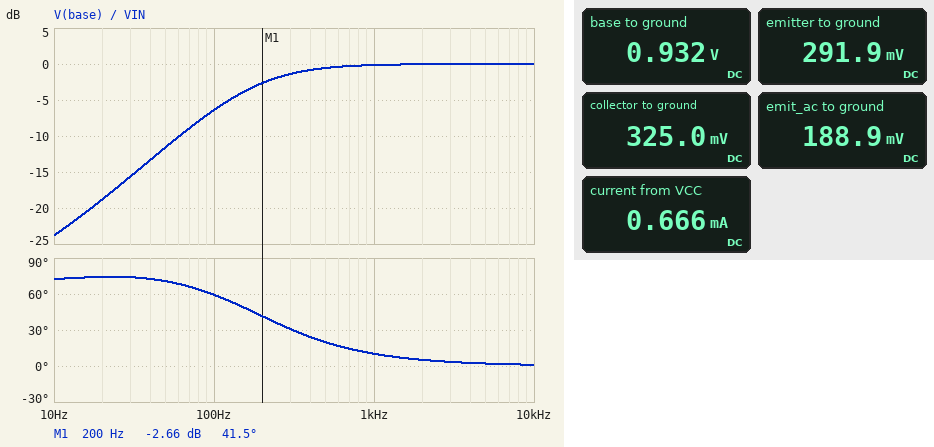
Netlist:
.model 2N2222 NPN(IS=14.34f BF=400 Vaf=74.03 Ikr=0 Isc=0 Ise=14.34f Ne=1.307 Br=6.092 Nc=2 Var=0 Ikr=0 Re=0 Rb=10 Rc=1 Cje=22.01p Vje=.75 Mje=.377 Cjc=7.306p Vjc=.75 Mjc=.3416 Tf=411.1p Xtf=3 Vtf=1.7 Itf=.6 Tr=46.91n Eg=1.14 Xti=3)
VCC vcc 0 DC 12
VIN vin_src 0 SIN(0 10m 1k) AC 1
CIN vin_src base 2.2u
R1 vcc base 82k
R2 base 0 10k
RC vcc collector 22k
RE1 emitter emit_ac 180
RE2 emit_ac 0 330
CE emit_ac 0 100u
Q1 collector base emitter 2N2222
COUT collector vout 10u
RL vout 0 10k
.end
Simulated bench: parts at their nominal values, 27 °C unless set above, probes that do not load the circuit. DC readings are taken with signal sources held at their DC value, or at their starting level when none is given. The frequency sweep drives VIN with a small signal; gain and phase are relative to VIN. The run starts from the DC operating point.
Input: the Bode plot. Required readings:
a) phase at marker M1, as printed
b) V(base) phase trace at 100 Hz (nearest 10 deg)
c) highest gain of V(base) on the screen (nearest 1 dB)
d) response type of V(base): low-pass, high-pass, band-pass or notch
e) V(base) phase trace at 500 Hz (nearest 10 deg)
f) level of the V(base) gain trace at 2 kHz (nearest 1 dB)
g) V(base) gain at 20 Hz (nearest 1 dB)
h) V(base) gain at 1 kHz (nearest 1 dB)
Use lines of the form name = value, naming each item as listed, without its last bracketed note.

phase at marker M1, as printed = 41.5 deg
V(base) phase trace at 100 Hz = 60 deg
highest gain of V(base) on the screen = 0 dB
response type of V(base): low-pass, high-pass, band-pass or notch = high-pass
V(base) phase trace at 500 Hz = 20 deg
level of the V(base) gain trace at 2 kHz = 0 dB
V(base) gain at 20 Hz = -19 dB
V(base) gain at 1 kHz = 0 dB
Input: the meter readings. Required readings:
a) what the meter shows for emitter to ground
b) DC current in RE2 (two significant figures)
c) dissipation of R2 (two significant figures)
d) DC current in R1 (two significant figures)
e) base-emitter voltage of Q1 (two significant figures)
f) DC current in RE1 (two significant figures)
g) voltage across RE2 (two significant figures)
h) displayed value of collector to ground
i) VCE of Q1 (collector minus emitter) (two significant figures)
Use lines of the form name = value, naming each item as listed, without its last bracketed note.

what the meter shows for emitter to ground = 291.9 mV
DC current in RE2 = 570 µA
dissipation of R2 = 87 µW
DC current in R1 = 130 µA
base-emitter voltage of Q1 = 640 mV
DC current in RE1 = 570 µA
voltage across RE2 = 190 mV
displayed value of collector to ground = 325.0 mV
VCE of Q1 (collector minus emitter) = 33 mV
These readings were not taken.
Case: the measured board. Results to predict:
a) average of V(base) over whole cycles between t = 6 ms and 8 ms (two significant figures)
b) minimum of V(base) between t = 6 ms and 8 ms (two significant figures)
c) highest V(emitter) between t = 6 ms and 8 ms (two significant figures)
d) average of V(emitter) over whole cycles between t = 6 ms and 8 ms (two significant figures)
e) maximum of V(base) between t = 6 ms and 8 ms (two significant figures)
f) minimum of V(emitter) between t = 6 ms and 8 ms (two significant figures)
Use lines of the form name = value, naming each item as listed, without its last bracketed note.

average of V(base) over whole cycles between t = 6 ms and 8 ms = 930 mV
minimum of V(base) between t = 6 ms and 8 ms = 920 mV
highest V(emitter) between t = 6 ms and 8 ms = 300 mV
average of V(emitter) over whole cycles between t = 6 ms and 8 ms = 290 mV
maximum of V(base) between t = 6 ms and 8 ms = 940 mV
minimum of V(emitter) between t = 6 ms and 8 ms = 290 mV
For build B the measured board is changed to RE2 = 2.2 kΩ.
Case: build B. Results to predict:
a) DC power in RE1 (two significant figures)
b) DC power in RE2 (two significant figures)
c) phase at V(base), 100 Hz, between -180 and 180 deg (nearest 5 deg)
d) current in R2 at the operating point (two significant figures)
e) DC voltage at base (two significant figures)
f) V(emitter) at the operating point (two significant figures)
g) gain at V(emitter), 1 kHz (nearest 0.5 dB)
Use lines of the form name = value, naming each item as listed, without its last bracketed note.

DC power in RE1 = 15 µW
DC power in RE2 = 180 µW
phase at V(base), 100 Hz, between -180 and 180 deg = 5 deg
current in R2 at the operating point = 130 µA
DC voltage at base = 1.3 V
V(emitter) at the operating point = 680 mV
gain at V(emitter), 1 kHz = -3.5 dB
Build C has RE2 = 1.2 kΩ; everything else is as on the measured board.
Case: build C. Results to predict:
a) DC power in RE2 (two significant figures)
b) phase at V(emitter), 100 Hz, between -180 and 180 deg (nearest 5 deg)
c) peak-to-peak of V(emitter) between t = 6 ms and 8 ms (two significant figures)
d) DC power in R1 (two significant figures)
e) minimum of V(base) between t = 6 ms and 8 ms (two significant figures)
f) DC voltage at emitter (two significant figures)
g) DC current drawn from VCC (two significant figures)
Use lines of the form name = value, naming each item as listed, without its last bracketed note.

DC power in RE2 = 270 µW
phase at V(emitter), 100 Hz, between -180 and 180 deg = 5 deg
peak-to-peak of V(emitter) between t = 6 ms and 8 ms = 15 mV
DC power in R1 = 1.4 mW
minimum of V(base) between t = 6 ms and 8 ms = 1.3 V
DC voltage at emitter = 650 mV
DC current drawn from VCC = 600 µA
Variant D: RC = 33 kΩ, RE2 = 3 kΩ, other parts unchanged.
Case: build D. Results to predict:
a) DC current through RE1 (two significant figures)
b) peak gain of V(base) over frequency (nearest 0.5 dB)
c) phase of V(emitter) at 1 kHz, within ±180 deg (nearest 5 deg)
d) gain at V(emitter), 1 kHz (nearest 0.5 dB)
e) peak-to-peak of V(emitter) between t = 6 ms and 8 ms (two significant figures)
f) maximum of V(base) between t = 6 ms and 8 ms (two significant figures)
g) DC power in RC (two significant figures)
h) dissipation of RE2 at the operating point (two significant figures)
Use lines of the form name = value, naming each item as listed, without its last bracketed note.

DC current through RE1 = 220 µA
peak gain of V(base) over frequency = 0 dB
phase of V(emitter) at 1 kHz, within ±180 deg = 0 deg
gain at V(emitter), 1 kHz = -4.5 dB
peak-to-peak of V(emitter) between t = 6 ms and 8 ms = 12 mV
maximum of V(base) between t = 6 ms and 8 ms = 1.3 V
DC power in RC = 1.5 mW
dissipation of RE2 at the operating point = 140 µW
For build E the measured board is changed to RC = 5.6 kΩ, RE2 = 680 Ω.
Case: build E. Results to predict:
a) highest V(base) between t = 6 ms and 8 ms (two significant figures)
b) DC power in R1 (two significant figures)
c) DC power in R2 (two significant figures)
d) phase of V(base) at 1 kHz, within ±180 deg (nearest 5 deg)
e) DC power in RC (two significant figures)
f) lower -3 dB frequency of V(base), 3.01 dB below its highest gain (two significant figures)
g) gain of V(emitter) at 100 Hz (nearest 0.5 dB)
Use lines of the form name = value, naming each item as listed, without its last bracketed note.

highest V(base) between t = 6 ms and 8 ms = 1.3 V
DC power in R1 = 1.4 mW
DC power in R2 = 160 µW
phase of V(base) at 1 kHz, within ±180 deg = 0 deg
DC power in RC = 3.0 mW
lower -3 dB frequency of V(base), 3.01 dB below its highest gain = 9.7 Hz
gain of V(emitter) at 100 Hz = -1.5 dB
